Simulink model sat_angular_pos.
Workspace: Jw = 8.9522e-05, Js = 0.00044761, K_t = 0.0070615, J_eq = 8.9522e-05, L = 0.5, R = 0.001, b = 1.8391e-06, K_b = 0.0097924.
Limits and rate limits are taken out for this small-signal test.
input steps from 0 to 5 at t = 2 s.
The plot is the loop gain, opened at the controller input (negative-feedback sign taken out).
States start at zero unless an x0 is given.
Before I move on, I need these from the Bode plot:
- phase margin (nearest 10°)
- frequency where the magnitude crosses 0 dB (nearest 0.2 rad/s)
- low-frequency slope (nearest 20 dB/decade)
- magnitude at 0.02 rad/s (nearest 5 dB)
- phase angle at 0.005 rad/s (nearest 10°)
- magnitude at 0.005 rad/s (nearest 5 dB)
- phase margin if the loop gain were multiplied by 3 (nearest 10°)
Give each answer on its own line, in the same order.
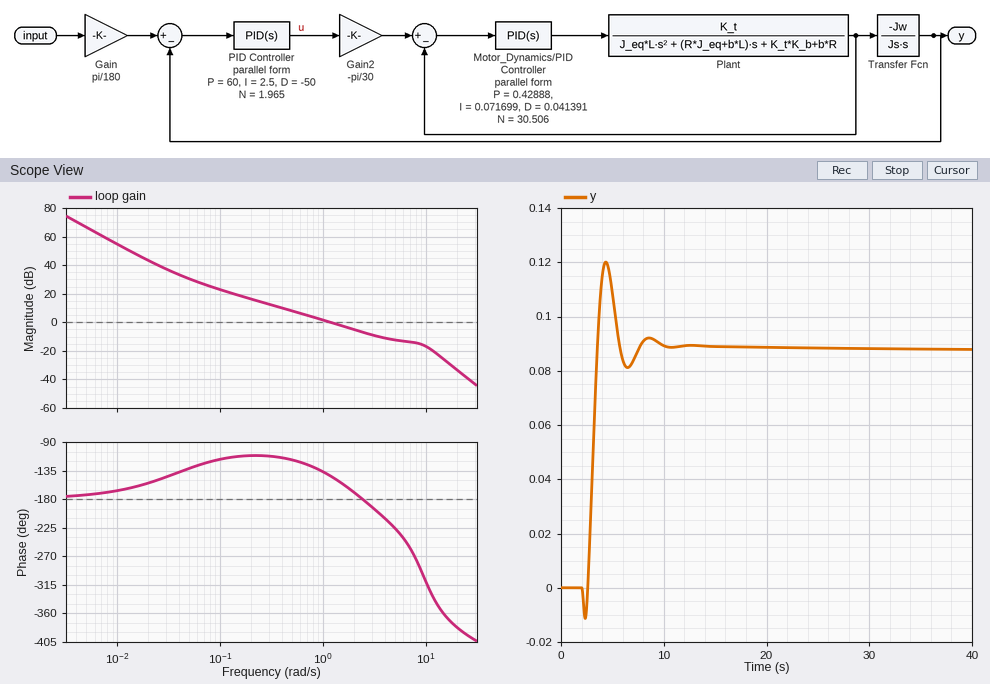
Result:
40°
1.2 rad/s
-40 dB/decade
45 dB
-170°
65 dB
-20°
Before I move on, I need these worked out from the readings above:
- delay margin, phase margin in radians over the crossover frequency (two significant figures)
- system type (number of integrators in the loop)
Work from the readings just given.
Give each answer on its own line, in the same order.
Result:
0.58 s
2
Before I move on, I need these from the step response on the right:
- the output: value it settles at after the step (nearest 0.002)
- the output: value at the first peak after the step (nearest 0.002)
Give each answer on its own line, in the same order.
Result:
0.088
0.120
